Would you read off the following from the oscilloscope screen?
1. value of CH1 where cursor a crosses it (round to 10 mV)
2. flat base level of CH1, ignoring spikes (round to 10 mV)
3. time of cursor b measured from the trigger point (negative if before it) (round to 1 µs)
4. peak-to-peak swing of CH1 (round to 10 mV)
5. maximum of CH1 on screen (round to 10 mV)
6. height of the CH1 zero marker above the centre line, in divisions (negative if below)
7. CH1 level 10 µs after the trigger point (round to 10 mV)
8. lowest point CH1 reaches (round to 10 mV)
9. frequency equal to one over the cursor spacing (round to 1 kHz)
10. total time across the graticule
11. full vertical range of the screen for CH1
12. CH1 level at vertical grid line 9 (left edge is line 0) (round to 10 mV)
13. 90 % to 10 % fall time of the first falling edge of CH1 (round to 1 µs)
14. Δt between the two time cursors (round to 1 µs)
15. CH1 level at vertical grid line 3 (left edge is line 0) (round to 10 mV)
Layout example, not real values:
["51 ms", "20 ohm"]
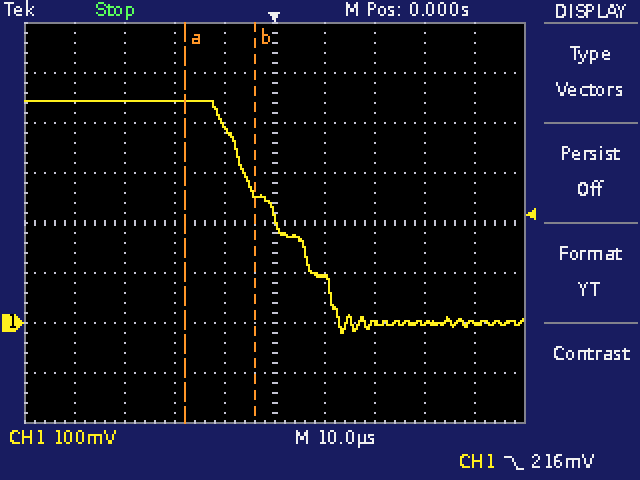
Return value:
["440 mV", "0 mV", "-4 µs", "460 mV", "440 mV", "-2.0 div", "90 mV", "-20 mV", "71 kHz", "100 µs", "800 mV", "0 mV", "22 µs", "14 µs", "440 mV"]
